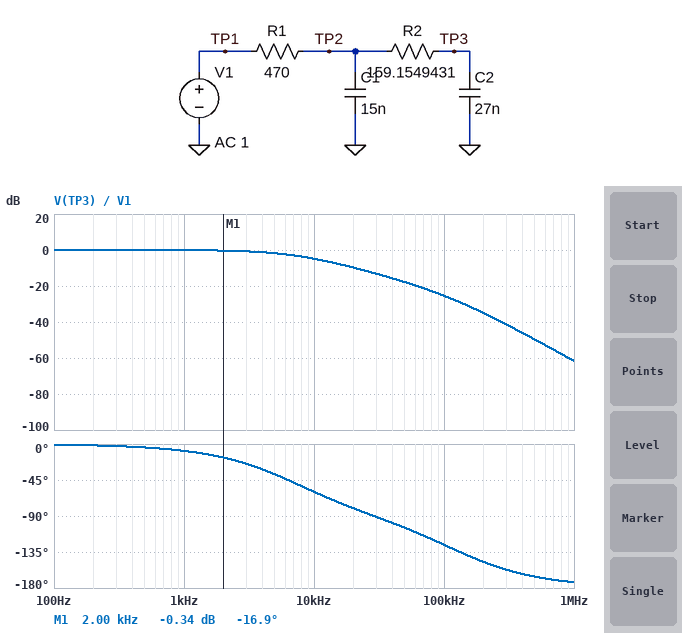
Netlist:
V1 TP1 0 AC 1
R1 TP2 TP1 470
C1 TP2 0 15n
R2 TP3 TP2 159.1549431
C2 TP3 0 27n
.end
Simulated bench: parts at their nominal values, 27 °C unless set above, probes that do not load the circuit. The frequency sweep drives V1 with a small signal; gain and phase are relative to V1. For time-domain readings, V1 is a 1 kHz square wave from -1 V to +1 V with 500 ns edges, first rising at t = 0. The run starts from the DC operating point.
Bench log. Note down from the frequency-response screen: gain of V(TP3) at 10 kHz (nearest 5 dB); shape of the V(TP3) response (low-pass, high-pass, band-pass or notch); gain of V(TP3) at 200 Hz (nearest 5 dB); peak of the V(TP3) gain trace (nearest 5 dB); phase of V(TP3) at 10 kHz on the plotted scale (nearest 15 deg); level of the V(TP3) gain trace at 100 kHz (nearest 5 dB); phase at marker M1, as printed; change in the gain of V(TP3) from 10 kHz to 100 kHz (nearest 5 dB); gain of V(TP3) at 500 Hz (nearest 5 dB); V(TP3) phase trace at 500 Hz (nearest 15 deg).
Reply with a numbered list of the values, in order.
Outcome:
1. -5 dB
2. low-pass
3. 0 dB
4. 0 dB
5. -60 deg
6. -25 dB
7. -16.9 deg
8. -20 dB
9. 0 dB
10. 0 deg
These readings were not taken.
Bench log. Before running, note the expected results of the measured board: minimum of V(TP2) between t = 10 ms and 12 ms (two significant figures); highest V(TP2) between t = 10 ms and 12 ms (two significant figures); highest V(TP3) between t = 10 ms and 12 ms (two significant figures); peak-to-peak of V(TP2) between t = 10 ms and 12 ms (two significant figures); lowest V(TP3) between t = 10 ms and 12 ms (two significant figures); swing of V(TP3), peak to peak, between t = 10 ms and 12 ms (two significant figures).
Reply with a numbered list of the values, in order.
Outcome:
1. -1.0 V
2. 1.0 V
3. 1.0 V
4. 2.0 V
5. -1.0 V
6. 2.0 V
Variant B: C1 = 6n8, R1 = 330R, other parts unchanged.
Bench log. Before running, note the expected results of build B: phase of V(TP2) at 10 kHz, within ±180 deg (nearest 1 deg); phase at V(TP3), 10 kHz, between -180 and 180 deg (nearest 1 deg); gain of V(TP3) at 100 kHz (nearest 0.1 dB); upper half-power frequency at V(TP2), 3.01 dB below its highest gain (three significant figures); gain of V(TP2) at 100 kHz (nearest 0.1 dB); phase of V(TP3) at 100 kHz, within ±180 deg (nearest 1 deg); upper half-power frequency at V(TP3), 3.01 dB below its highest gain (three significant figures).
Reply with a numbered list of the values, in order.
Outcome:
1. -30 deg
2. -45 deg
3. -20.1 dB
4. 11.8 kHz
5. -10.9 dB
6. -106 deg
7. 10.7 kHz
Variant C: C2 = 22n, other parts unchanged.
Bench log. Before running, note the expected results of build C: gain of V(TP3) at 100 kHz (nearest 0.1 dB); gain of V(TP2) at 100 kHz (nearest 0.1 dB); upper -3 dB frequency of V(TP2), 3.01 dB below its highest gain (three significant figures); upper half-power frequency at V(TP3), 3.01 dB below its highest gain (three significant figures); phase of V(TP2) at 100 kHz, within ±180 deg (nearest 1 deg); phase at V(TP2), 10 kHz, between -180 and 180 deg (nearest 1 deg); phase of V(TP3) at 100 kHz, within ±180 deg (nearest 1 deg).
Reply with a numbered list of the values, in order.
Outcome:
1. -24.0 dB
2. -16.3 dB
3. 8.34 kHz
4. 8.07 kHz
5. -58 deg
6. -43 deg
7. -124 deg
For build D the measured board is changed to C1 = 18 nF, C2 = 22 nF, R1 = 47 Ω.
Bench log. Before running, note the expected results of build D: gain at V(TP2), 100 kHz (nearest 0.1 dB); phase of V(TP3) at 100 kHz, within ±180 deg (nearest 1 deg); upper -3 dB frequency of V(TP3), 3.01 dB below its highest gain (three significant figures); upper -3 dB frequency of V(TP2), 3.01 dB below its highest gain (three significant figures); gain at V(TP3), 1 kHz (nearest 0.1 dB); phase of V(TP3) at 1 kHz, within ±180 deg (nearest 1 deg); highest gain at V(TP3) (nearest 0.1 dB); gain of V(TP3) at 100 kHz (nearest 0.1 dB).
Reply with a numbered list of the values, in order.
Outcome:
1. -2.9 dB
2. -93 deg
3. 32.9 kHz
4. 105 kHz
5. 0 dB
6. -2 deg
7. 0 dB
8. -10.6 dB
